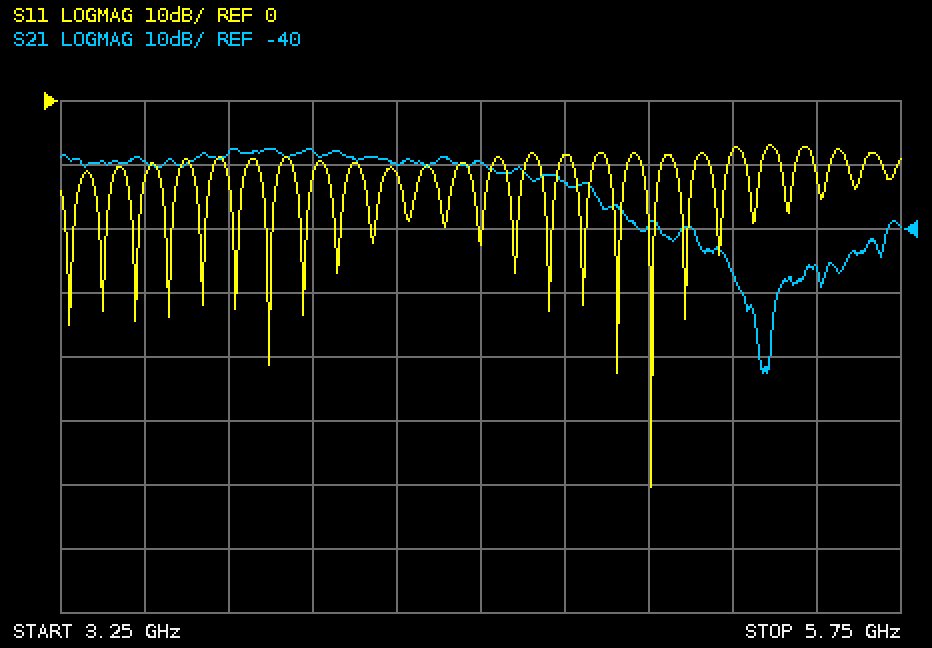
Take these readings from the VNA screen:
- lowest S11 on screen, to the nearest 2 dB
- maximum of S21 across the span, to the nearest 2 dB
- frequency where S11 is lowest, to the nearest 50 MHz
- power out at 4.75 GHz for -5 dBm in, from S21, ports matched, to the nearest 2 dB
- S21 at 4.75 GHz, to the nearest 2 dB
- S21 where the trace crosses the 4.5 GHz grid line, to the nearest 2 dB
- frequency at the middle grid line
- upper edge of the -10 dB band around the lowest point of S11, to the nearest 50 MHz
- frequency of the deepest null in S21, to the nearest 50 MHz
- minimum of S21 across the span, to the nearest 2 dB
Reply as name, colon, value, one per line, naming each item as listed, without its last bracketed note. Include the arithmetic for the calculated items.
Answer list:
lowest S11 on screen, to the nearest 2 dB: -60 dB
maximum of S21 across the span, to the nearest 2 dB: -28 dB
frequency where S11 is lowest, to the nearest 50 MHz: 5.00 GHz
power out at 4.75 GHz for -5 dBm in, from S21, ports matched, to the nearest 2 dB: -5 dBm + (-32 dB) = -38 dBm
S21 at 4.75 GHz, to the nearest 2 dB: -32 dB
S21 where the trace crosses the 4.5 GHz grid line, to the nearest 2 dB: -30 dB
frequency at the middle grid line: 4.5 GHz
upper edge of the -10 dB band around the lowest point of S11, to the nearest 50 MHz: 5.05 GHz
frequency of the deepest null in S21, to the nearest 50 MHz: 5.35 GHz
minimum of S21 across the span, to the nearest 2 dB: -62 dB
